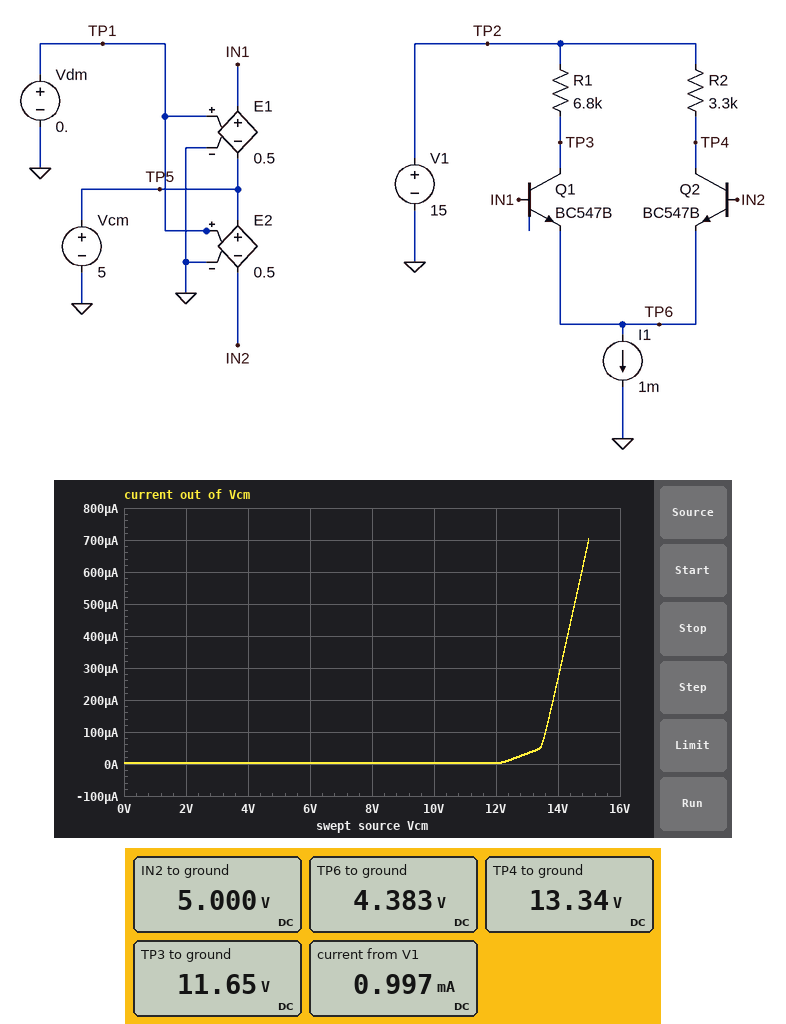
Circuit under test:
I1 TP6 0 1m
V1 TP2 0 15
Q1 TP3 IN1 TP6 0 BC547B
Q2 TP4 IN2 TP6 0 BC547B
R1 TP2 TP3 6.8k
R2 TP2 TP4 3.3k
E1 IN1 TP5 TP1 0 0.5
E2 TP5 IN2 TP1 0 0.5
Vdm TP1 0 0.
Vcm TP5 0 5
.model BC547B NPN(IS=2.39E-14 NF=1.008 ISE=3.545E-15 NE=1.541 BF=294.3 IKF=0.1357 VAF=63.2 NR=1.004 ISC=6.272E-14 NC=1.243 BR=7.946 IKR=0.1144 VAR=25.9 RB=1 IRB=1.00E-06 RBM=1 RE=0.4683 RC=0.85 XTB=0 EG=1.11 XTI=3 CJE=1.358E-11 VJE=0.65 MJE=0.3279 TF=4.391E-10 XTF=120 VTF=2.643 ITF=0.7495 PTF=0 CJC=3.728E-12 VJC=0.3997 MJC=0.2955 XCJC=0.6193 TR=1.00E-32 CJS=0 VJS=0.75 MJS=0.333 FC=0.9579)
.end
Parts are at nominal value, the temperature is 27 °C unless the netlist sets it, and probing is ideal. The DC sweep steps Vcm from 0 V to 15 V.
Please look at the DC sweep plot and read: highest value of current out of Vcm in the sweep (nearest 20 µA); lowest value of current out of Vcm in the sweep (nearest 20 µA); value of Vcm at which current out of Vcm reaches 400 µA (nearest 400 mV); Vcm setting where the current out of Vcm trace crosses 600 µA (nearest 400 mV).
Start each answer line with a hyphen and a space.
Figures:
- 700 µA
- 0 A
- 14.4 V
- 14.8 V
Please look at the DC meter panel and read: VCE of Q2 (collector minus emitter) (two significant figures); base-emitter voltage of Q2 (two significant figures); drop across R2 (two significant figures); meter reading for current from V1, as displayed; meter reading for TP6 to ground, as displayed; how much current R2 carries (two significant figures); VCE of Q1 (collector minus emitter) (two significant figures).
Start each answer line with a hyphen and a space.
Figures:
- 9.0 V
- 620 mV
- 1.7 V
- 0.997 mA
- 4.383 V
- 500 µA
- 7.3 V
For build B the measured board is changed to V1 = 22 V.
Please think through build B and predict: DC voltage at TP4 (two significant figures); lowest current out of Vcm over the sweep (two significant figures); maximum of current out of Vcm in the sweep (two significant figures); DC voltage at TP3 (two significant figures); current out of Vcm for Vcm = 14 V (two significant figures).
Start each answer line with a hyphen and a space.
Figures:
- 20 V
- 2.7 µA
- 3.3 µA
- 19 V
- 3.2 µA
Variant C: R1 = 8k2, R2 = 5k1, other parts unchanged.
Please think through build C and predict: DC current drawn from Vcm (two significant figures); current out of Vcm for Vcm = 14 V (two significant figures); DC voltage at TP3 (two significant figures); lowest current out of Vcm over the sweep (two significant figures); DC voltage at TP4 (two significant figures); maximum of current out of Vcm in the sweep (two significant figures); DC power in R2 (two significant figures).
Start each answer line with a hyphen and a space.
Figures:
- 3.2 µA
- 480 µA
- 11 V
- 3.0 µA
- 12 V
- 790 µA
- 1.3 mW
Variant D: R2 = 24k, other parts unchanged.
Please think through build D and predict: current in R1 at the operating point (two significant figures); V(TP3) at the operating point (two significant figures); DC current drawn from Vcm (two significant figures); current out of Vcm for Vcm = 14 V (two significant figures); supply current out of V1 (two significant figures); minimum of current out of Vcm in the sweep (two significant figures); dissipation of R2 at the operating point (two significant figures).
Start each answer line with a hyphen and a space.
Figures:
- 550 µA
- 11 V
- 12 µA
- 690 µA
- 990 µA
- 3.1 µA
- 4.6 mW
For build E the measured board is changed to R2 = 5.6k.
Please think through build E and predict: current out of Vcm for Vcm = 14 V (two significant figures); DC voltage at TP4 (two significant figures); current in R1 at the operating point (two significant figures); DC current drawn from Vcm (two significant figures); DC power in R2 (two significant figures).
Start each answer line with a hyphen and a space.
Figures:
- 460 µA
- 12 V
- 500 µA
- 3.2 µA
- 1.4 mW
